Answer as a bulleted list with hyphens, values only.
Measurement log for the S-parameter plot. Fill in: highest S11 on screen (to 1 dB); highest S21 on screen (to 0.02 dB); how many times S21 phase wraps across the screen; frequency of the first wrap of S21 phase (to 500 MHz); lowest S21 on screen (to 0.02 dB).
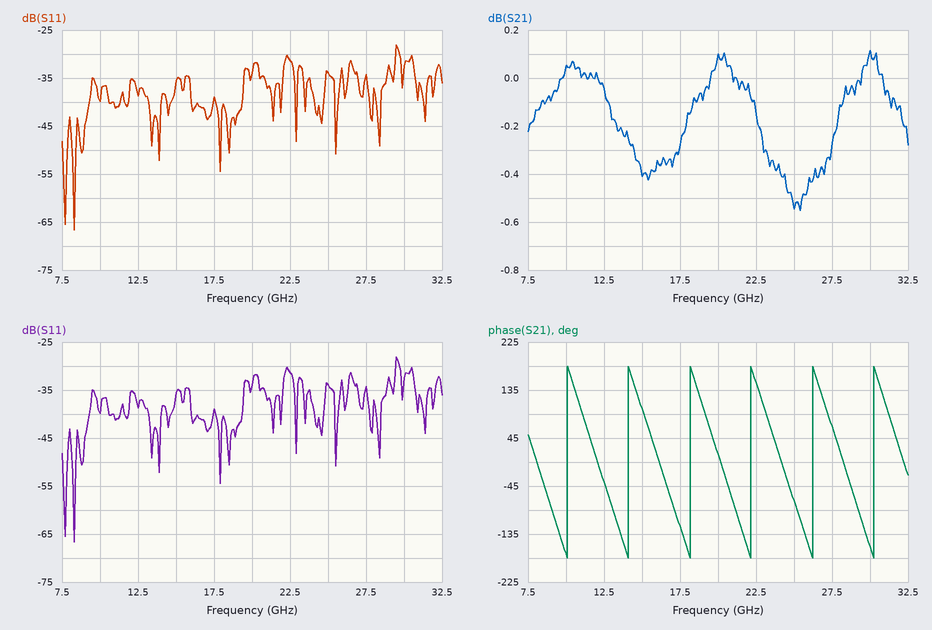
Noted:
- -28 dB
- 0.12 dB
- 6
- 10.0 GHz
- -0.56 dB
